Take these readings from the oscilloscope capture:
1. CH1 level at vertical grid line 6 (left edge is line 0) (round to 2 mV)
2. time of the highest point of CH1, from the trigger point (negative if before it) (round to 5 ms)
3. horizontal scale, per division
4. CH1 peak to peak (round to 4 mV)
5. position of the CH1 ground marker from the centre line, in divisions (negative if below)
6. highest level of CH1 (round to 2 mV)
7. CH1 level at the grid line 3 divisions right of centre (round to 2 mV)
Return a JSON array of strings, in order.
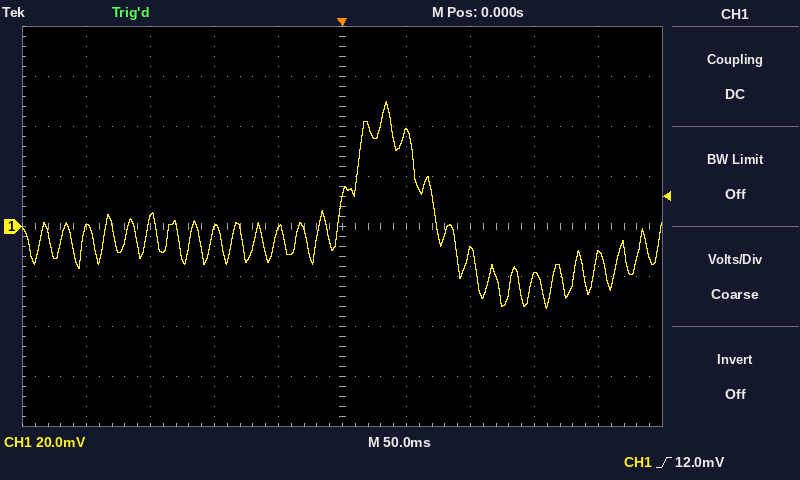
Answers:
["38 mV", "+35 ms", "50 ms", "84 mV", "0.0 div", "50 mV", "-20 mV"]
